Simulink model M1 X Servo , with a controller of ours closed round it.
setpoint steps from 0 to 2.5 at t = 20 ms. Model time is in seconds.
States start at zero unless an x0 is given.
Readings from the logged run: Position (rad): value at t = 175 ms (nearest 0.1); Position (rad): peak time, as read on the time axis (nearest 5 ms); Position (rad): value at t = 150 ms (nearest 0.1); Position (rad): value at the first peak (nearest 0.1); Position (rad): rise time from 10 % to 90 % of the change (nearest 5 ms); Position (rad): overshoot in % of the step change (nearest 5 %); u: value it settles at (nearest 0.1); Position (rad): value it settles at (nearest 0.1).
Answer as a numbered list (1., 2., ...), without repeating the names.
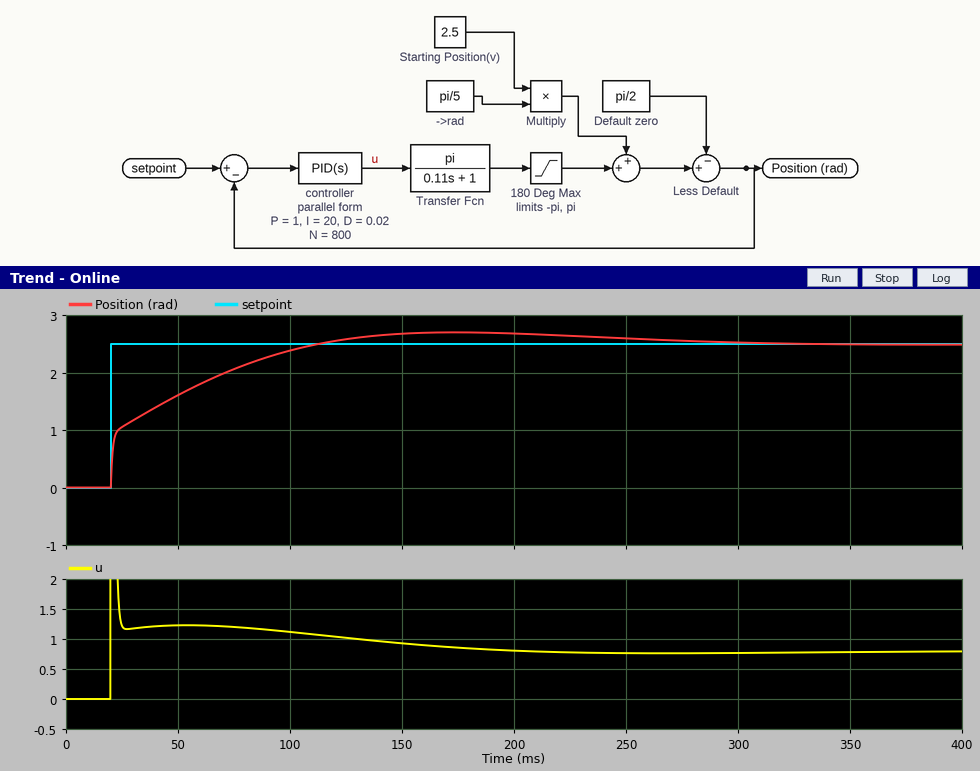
1. 2.7
2. 175 ms
3. 2.7
4. 2.7
5. 70 ms
6. 10 %
7. 0.8
8. 2.5
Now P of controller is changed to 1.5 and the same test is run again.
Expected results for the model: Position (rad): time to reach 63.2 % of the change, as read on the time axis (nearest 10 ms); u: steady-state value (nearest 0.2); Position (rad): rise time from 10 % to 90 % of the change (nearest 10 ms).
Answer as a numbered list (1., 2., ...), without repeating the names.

1. 40 ms
2. 0.8
3. 60 ms
